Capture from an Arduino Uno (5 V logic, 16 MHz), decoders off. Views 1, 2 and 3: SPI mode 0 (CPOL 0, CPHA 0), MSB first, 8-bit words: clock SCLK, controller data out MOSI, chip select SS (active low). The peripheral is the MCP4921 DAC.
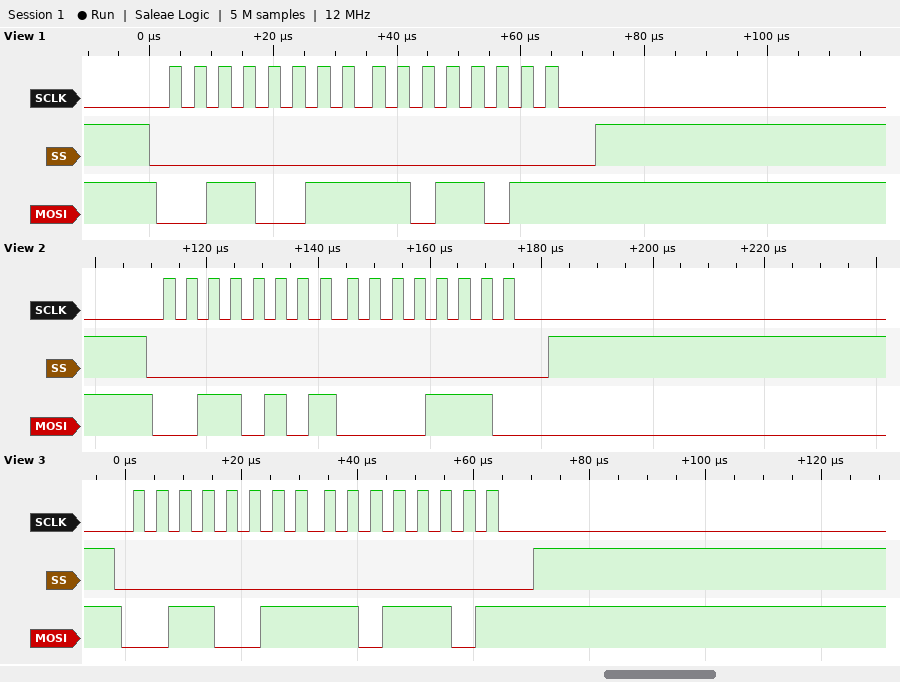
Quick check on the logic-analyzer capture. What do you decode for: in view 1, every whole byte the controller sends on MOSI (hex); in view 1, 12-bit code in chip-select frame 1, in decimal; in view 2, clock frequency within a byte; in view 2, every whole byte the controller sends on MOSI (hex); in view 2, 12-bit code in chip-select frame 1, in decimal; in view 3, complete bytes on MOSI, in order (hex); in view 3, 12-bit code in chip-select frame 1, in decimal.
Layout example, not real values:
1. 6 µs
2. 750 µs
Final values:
1. 33 DB
2. 987
3. 250 kHz
4. 35 0E
5. 1294
6. 33 DD
7. 989
